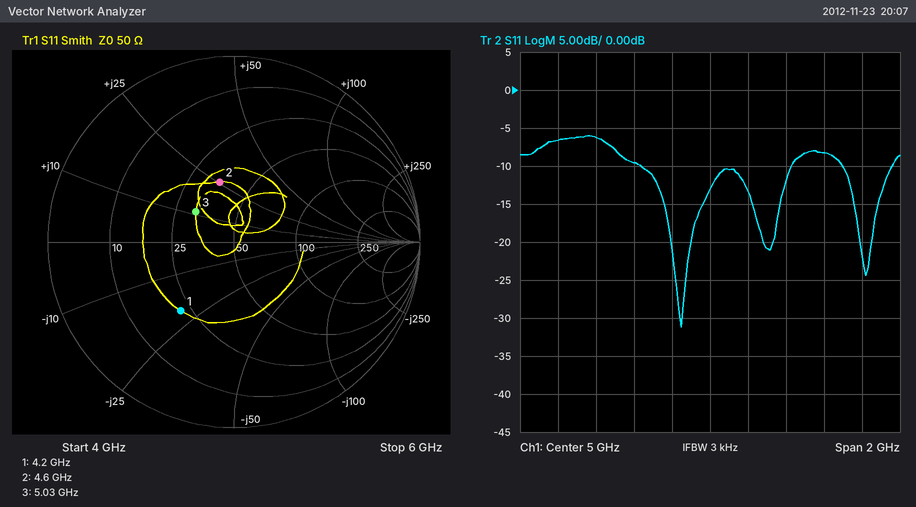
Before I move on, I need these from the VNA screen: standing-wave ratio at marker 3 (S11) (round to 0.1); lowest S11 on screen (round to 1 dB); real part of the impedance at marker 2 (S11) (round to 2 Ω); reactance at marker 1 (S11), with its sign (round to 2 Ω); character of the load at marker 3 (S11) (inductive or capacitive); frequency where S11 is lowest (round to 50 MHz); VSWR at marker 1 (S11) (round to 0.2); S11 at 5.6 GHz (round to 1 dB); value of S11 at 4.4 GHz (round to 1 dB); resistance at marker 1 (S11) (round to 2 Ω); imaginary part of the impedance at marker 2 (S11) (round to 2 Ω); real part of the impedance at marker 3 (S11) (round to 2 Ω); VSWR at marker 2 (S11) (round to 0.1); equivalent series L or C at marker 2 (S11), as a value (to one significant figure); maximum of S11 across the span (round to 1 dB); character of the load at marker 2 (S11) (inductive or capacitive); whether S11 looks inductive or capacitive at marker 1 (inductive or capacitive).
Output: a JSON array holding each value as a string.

["1.7", "-31 dB", "36 Ω", "-20 Ω", "inductive", "4.85 GHz", "2.8", "-8 dB", "-6 dB", "22 Ω", "+26 Ω", "32 Ω", "2.0", "900 pH", "-6 dB", "inductive", "capacitive"]
